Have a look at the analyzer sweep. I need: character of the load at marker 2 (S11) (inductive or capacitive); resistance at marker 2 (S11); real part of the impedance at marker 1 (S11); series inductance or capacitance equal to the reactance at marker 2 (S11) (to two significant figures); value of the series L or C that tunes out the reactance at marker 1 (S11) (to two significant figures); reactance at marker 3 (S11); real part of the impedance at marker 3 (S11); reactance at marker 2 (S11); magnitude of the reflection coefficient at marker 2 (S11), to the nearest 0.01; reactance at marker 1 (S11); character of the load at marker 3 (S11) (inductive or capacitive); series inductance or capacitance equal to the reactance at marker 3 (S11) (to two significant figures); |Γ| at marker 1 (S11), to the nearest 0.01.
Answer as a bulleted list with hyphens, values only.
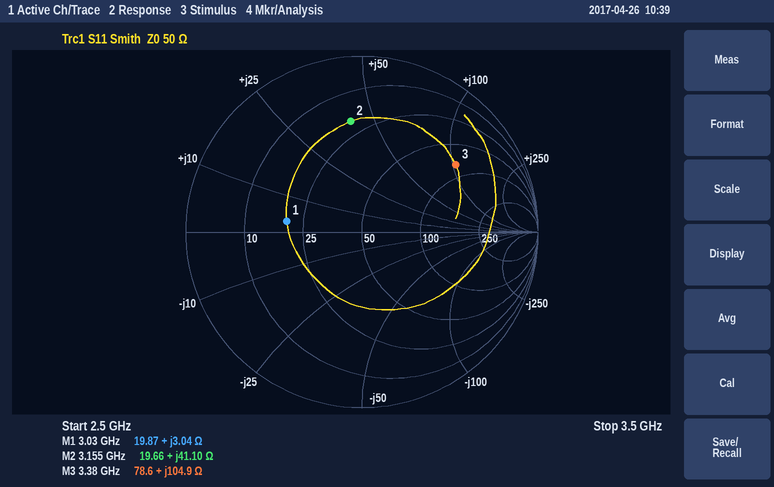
- inductive
- 19.66 Ω
- 19.87 Ω
- 2.1 nH
- 17 pF
- +104.9 Ω
- 78.6 Ω
- +41.10 Ω
- 0.63
- +3.04 Ω
- inductive
- 4.9 nH
- 0.43
